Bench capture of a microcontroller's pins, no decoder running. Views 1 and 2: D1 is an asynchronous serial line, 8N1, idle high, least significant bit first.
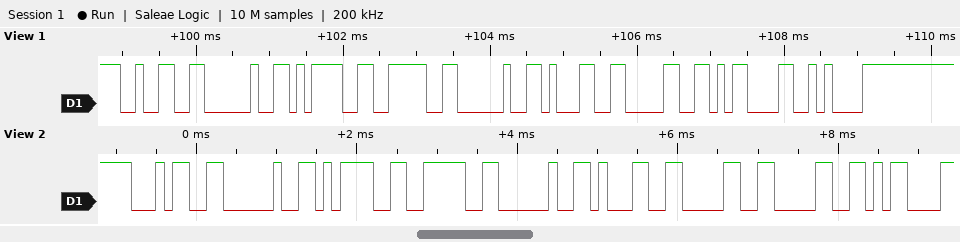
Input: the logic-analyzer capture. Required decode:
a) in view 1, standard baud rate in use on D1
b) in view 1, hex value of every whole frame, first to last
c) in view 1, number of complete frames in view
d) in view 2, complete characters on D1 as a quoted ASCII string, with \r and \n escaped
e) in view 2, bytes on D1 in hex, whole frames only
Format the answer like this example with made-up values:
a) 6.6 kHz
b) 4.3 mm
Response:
a) 9600 baud
b) 32 20 3D 3E 20 31 30 0D 0A
c) 9
d) "4 => 100\r"
e) 0x34 0x20 0x3D 0x3E 0x20 0x31 0x30 0x30 0x0D
